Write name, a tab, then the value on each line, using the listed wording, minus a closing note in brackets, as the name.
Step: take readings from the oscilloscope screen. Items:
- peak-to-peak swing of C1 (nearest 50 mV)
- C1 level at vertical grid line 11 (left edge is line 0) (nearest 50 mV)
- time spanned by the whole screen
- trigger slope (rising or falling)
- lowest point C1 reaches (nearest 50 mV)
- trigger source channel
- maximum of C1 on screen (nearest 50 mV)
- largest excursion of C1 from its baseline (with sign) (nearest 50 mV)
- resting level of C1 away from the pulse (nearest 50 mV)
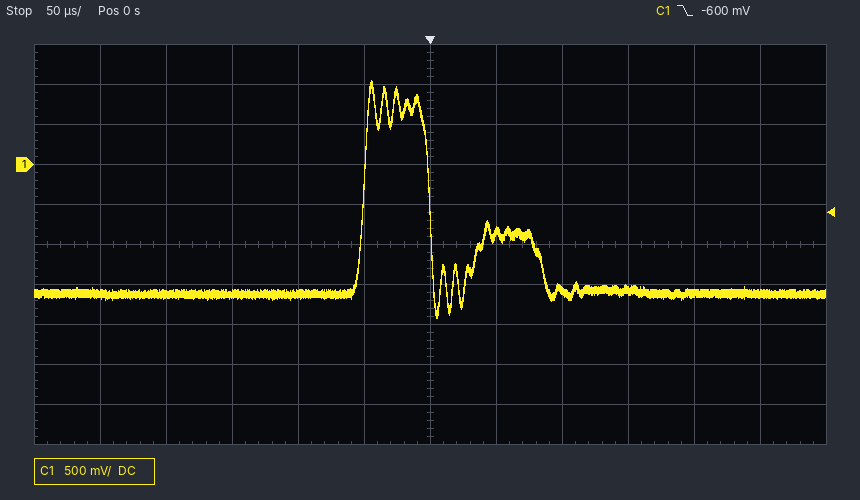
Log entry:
peak-to-peak swing of C1	2.95 V
C1 level at vertical grid line 11 (left edge is line 0)	-1.60 V
time spanned by the whole screen	600 µs
trigger slope	falling
lowest point C1 reaches	-1.90 V
trigger source channel	C1
maximum of C1 on screen	1.05 V
largest excursion of C1 from its baseline (with sign)	+2.65 V
resting level of C1 away from the pulse	-1.60 V
